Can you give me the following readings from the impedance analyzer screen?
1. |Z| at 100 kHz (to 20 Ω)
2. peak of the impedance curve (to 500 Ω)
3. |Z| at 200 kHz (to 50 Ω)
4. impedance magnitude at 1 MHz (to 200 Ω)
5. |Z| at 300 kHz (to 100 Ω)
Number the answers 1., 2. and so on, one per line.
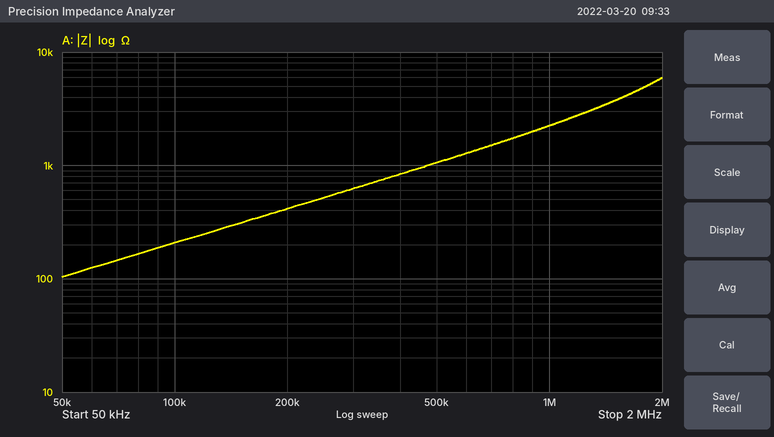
1. 200 Ω
2. 6.0 kΩ
3. 400 Ω
4. 2.2 kΩ
5. 600 Ω
